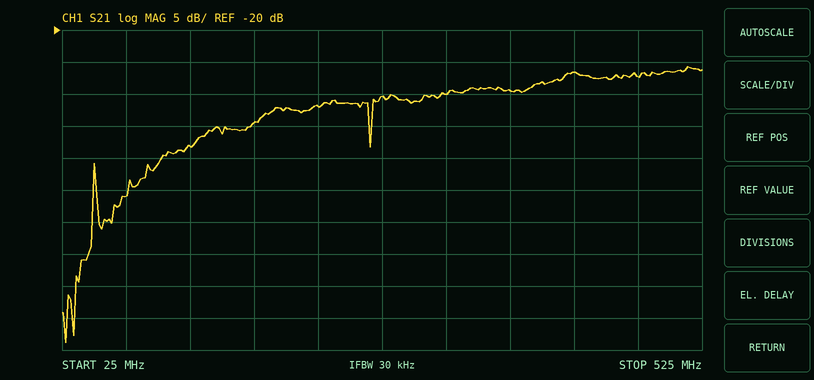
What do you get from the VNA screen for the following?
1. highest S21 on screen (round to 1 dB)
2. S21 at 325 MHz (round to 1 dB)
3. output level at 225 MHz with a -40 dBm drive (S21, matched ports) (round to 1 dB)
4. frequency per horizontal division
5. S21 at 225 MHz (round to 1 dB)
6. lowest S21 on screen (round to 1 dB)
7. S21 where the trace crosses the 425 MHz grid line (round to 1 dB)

-26 dB
-30 dB
-72 dBm
50 MHz
-32 dB
-69 dB
-27 dB
